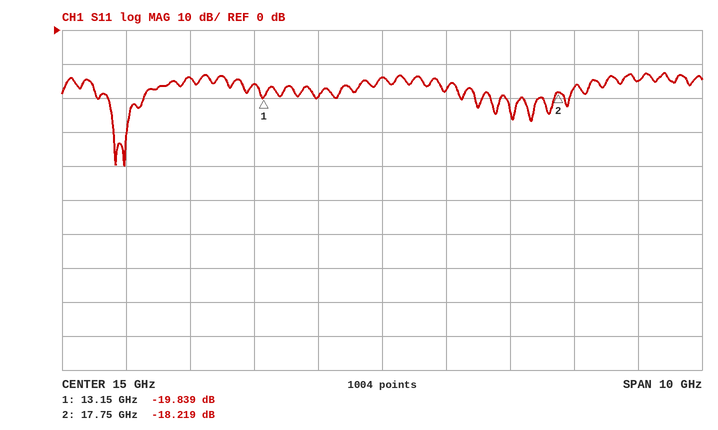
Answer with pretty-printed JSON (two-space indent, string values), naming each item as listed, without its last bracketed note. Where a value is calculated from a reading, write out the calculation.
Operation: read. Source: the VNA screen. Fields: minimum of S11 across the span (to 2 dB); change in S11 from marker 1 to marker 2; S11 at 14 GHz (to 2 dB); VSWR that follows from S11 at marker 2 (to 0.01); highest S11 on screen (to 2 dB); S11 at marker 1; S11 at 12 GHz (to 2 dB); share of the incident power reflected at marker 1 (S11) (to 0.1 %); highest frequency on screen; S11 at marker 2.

{
  "minimum of S11 across the span": "-40 dB",
  "change in S11 from marker 1 to marker 2": "-18.219 − (-19.839) = 1.620 dB",
  "S11 at 14 GHz": "-20 dB",
  "VSWR that follows from S11 at marker 2": "(1 + 0.1228)/(1 − 0.1228) ≈ 1.28",
  "highest S11 on screen": "-12 dB",
  "S11 at marker 1": "-19.839 dB",
  "S11 at 12 GHz": "-14 dB",
  "share of the incident power reflected at marker 1 (S11)": "10^(-19.839/10) ≈ 1.0 %",
  "highest frequency on screen": "20 GHz",
  "S11 at marker 2": "-18.219 dB"
}
